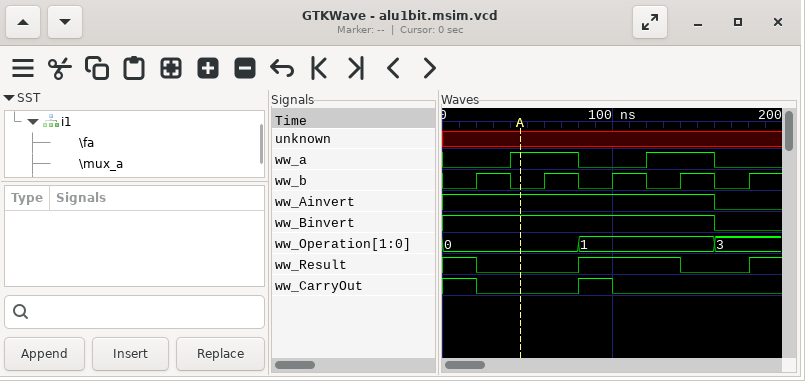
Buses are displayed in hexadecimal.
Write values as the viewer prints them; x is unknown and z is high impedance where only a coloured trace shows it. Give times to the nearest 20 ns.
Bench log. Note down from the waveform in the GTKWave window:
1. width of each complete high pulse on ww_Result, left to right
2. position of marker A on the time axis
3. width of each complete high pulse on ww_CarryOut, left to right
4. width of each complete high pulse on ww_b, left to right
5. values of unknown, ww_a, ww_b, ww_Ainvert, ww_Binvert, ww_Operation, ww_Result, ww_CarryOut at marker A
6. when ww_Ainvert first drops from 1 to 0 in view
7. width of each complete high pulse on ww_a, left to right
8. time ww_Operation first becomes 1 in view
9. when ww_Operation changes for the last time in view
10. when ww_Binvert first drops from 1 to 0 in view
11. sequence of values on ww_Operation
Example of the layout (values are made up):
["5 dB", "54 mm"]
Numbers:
["60 ns", "40 ns", "20 ns", "20 ns, 20 ns, 20 ns, 20 ns", "unknown=x, ww_a=1, ww_b=0, ww_Ainvert=1, ww_Binvert=1, ww_Operation=0, ww_Result=0, ww_CarryOut=0", "160 ns", "40 ns, 40 ns", "80 ns", "160 ns", "160 ns", "0, 1, 3"]
